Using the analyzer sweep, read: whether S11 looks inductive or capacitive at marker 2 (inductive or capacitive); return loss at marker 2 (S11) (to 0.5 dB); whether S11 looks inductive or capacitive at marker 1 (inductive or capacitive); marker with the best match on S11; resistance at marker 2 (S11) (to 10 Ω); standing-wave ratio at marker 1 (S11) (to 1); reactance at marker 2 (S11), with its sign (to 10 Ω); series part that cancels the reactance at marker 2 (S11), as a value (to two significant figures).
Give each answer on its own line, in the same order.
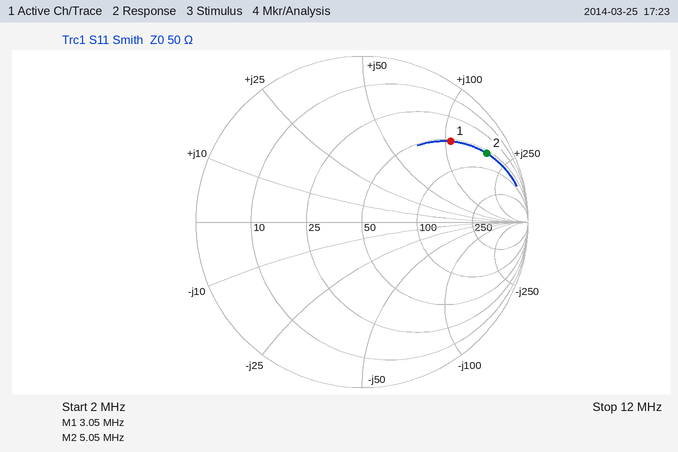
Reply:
inductive
1.5 dB
inductive
marker 1
60 Ω
6
+180 Ω
180 pF
